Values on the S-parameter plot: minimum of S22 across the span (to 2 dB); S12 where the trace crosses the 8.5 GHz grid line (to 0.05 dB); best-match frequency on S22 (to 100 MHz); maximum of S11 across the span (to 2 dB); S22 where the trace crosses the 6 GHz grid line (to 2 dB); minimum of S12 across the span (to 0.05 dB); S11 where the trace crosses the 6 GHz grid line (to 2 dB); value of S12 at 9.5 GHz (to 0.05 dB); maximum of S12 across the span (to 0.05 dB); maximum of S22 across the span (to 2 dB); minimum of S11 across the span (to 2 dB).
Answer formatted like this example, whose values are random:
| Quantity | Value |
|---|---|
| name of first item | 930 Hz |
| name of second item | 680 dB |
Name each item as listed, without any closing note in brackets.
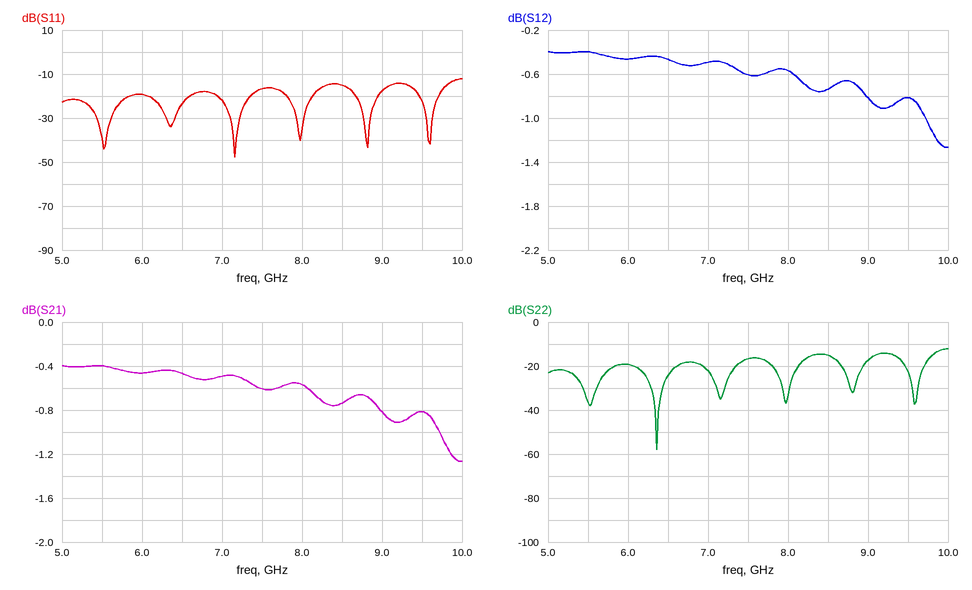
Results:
| Quantity | Value |
|---|---|
| minimum of S22 across the span | -58 dB |
| S12 where the trace crosses the 8.5 GHz grid line | -0.75 dB |
| best-match frequency on S22 | 6.4 GHz |
| maximum of S11 across the span | -12 dB |
| S22 where the trace crosses the 6 GHz grid line | -20 dB |
| minimum of S12 across the span | -1.25 dB |
| S11 where the trace crosses the 6 GHz grid line | -20 dB |
| value of S12 at 9.5 GHz | -0.80 dB |
| maximum of S12 across the span | -0.40 dB |
| maximum of S22 across the span | -12 dB |
| minimum of S11 across the span | -48 dB |
